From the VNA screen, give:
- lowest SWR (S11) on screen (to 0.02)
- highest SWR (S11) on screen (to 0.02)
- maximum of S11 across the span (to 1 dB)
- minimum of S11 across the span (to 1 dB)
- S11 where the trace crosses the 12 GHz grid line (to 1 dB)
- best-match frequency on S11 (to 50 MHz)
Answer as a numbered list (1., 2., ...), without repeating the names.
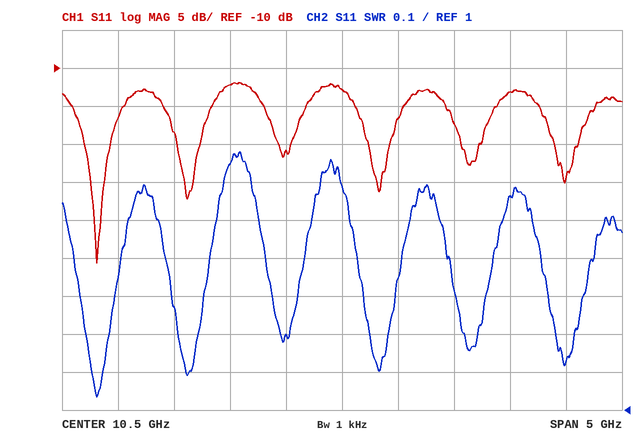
1. 1.04
2. 1.68
3. -12 dB
4. -36 dB
5. -13 dB
6. 8.30 GHz
